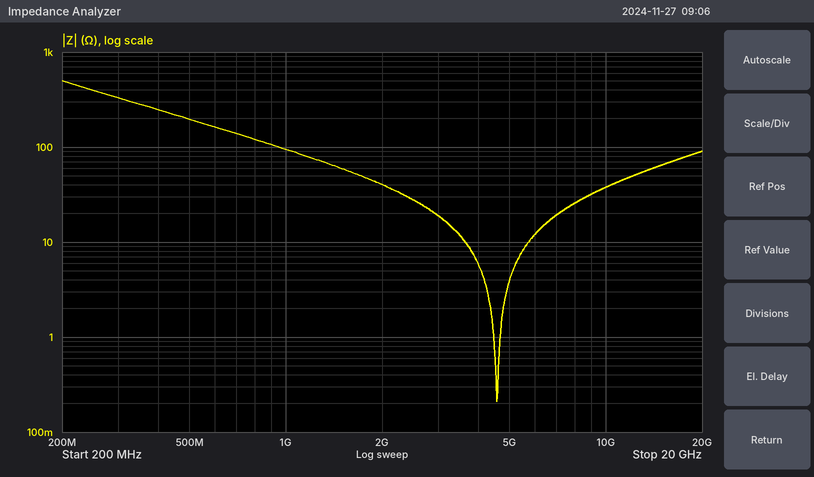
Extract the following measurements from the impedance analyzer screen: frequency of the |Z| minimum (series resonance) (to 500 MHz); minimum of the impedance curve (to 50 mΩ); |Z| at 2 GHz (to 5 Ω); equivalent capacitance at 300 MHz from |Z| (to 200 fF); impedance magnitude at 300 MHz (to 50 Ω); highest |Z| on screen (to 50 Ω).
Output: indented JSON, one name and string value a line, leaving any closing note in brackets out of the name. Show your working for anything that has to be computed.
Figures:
{
  "frequency of the |Z| minimum (series resonance)": "4.5 GHz",
  "minimum of the impedance curve": "200 mΩ",
  "|Z| at 2 GHz": "40 Ω",
  "equivalent capacitance at 300 MHz from |Z|": "C = 1/(2π × 300 MHz × 350 Ω) ≈ 1.52 pF, so 1.6 pF to the nearest 200 fF",
  "impedance magnitude at 300 MHz": "350 Ω",
  "highest |Z| on screen": "500 Ω"
}
